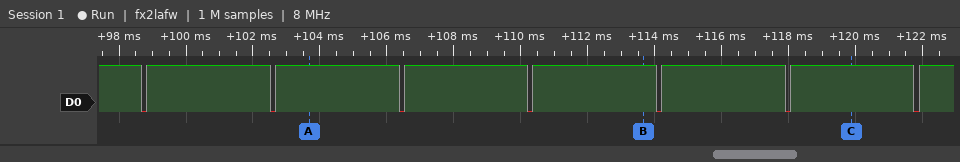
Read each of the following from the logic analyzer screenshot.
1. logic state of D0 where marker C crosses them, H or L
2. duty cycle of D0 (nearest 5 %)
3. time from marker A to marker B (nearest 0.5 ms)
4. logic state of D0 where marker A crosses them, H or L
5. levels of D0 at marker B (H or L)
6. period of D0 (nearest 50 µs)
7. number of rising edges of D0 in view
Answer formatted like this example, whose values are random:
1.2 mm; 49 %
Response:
D0=H; 95 %; 10 ms; D0=H; D0=H; 3850 µs; 7
